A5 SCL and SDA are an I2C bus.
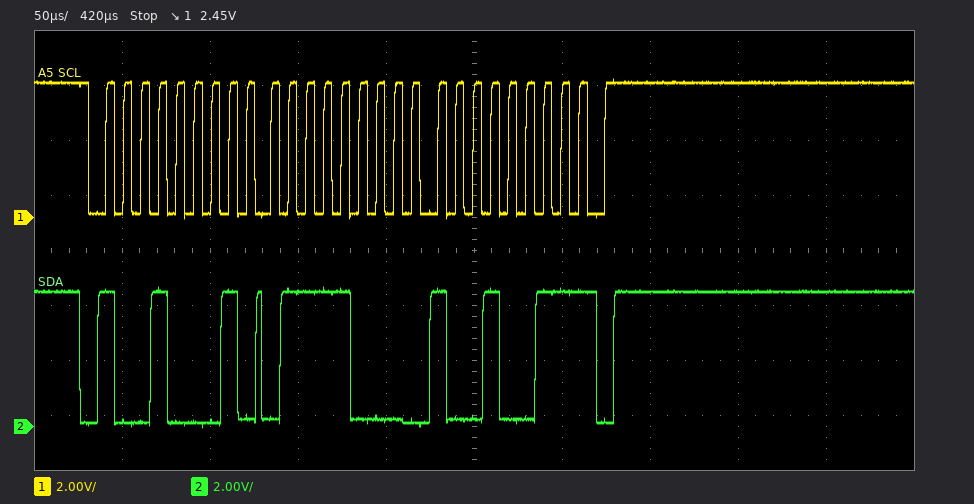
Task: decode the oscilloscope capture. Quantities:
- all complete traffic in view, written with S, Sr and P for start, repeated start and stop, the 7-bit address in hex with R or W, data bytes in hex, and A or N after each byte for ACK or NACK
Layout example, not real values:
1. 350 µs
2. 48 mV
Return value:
1. S 48R A 78 A 93 N P
